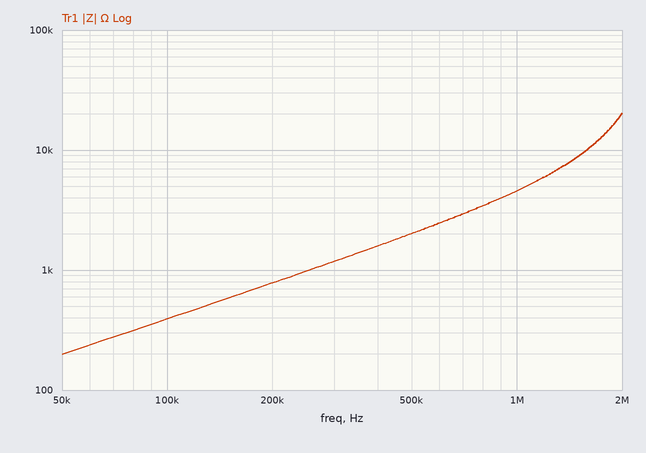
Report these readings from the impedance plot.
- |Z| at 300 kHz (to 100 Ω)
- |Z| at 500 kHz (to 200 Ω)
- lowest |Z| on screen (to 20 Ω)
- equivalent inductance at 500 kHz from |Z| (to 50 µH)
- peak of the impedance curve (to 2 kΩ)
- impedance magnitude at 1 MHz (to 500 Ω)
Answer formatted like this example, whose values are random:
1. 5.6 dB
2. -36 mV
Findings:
1. 1.2 kΩ
2. 2.0 kΩ
3. 200 Ω
4. 650 µH
5. 20 kΩ
6. 4.5 kΩ
